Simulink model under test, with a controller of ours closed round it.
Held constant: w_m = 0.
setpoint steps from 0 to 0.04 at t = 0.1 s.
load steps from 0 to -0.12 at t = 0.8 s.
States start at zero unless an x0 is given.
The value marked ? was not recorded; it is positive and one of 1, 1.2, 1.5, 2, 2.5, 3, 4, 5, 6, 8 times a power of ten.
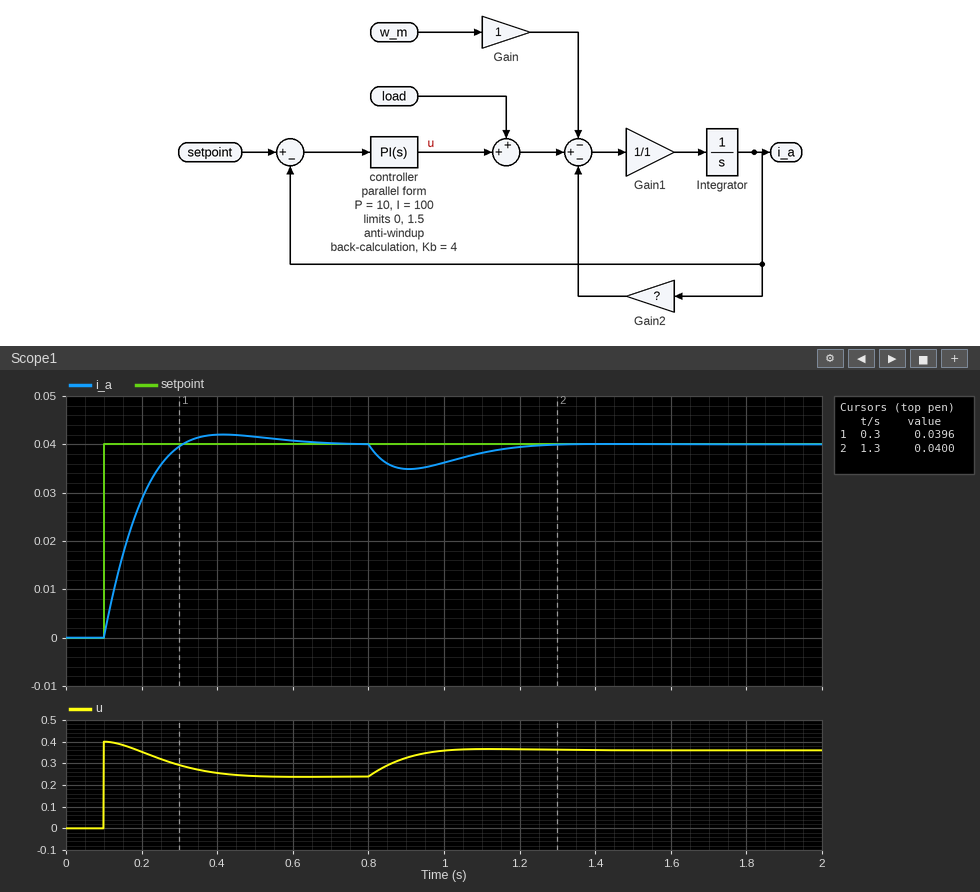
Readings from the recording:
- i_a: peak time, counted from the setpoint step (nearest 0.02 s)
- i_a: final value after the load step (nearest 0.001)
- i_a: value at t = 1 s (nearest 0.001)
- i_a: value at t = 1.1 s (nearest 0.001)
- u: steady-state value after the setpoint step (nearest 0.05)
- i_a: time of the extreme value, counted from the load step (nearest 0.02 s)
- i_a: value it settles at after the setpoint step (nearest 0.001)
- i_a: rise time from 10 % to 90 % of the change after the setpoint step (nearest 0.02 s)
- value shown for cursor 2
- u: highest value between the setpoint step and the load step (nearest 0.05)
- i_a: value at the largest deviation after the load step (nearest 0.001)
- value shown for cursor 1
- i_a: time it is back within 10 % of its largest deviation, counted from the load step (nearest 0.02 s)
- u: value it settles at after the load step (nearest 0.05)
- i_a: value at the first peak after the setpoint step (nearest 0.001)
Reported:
0.32 s
0.040
0.036
0.038
0.25
0.10 s
0.040
0.14 s
0.0400
0.40
0.035
0.0396
0.40 s
0.35
0.042
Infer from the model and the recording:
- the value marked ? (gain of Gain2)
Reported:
6
